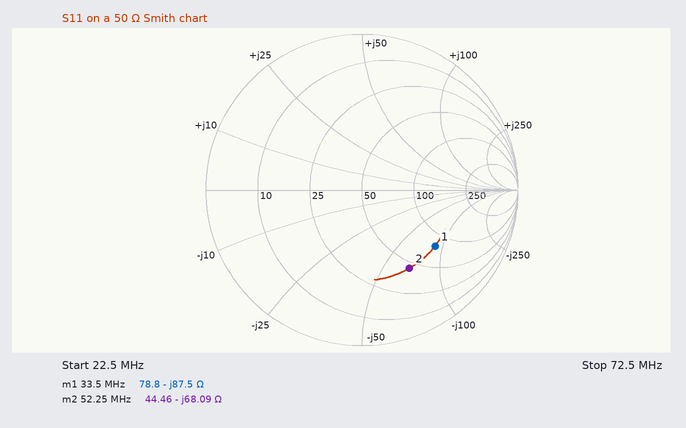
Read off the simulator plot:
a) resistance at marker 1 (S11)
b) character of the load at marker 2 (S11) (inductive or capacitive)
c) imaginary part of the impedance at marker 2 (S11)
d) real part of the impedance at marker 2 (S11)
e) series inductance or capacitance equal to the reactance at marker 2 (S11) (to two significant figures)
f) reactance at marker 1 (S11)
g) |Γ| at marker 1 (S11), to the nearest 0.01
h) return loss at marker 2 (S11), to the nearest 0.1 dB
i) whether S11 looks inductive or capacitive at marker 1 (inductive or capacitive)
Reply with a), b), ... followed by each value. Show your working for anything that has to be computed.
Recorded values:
a) 78.8 Ω
b) capacitive
c) -68.09 Ω
d) 44.46 Ω
e) C = 1/(2π × 52.25 MHz × 68.09 Ω) ≈ 45 pF
f) -87.5 Ω
g) 0.59
h) 4.6 dB
i) capacitive
